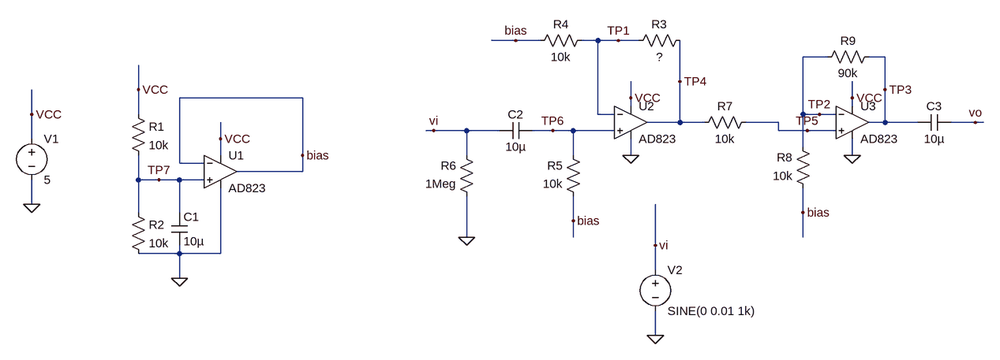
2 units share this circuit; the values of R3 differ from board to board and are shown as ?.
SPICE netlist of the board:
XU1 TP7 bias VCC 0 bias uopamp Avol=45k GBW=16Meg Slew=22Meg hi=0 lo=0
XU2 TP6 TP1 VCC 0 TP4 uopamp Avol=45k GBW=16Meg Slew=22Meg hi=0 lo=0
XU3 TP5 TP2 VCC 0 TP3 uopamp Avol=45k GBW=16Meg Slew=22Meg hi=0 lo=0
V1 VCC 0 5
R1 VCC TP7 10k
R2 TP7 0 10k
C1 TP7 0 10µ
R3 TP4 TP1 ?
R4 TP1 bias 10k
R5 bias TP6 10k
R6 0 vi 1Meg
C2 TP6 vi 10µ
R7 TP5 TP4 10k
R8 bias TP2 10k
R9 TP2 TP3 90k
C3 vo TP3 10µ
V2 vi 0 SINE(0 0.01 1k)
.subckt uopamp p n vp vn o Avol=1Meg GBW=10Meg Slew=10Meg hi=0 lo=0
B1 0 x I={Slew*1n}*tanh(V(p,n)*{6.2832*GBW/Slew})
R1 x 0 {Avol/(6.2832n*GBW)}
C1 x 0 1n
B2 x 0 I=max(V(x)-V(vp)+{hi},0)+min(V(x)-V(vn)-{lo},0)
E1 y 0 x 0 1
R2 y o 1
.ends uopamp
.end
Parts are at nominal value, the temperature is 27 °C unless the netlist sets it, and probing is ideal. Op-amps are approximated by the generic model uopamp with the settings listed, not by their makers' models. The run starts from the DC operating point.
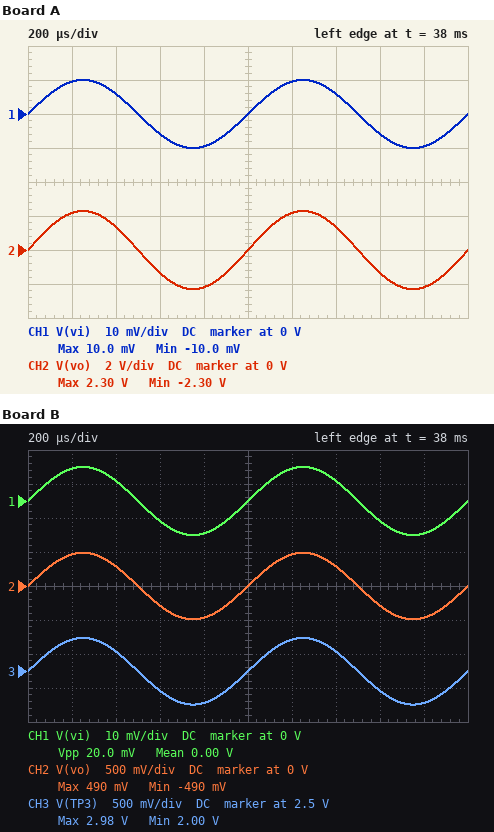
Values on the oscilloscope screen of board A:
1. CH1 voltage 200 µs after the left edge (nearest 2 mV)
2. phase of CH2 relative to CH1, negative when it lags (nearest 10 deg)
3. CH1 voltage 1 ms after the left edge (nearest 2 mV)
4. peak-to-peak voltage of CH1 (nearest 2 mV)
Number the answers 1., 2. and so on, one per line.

1. 10 mV
2. 0 deg
3. 0 V
4. 20 mV
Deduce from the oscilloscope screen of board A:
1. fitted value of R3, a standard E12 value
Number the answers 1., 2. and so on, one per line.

1. 220 kΩ
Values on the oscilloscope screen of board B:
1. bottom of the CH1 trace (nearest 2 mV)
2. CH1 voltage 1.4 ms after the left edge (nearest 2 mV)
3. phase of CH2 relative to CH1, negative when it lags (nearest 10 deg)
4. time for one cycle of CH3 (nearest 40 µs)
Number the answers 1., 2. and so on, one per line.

1. -10 mV
2. 6 mV
3. 0 deg
4. 1.00 ms
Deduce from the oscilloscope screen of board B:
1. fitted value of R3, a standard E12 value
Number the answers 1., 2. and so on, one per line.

1. 39 kΩ
